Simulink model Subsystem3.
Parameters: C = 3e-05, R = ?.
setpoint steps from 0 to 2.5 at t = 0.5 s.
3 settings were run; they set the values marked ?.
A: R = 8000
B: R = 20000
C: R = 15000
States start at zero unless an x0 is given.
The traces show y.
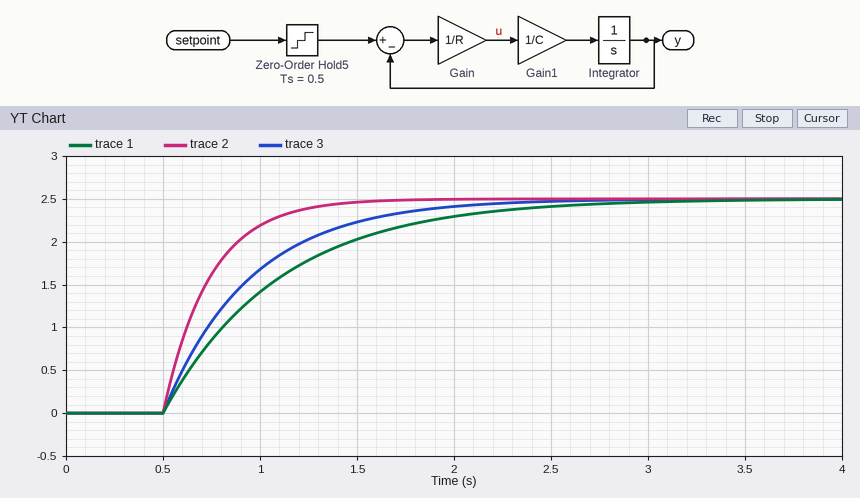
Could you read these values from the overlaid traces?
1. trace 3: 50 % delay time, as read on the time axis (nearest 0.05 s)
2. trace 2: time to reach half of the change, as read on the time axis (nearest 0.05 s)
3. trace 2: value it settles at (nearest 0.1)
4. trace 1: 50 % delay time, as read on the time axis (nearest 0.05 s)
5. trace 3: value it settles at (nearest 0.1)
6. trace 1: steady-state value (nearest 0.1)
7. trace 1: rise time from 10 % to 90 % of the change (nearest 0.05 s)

0.80 s
0.65 s
2.5
0.90 s
2.5
2.5
1.30 s
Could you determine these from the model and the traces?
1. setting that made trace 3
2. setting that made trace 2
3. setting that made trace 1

C
A
B
